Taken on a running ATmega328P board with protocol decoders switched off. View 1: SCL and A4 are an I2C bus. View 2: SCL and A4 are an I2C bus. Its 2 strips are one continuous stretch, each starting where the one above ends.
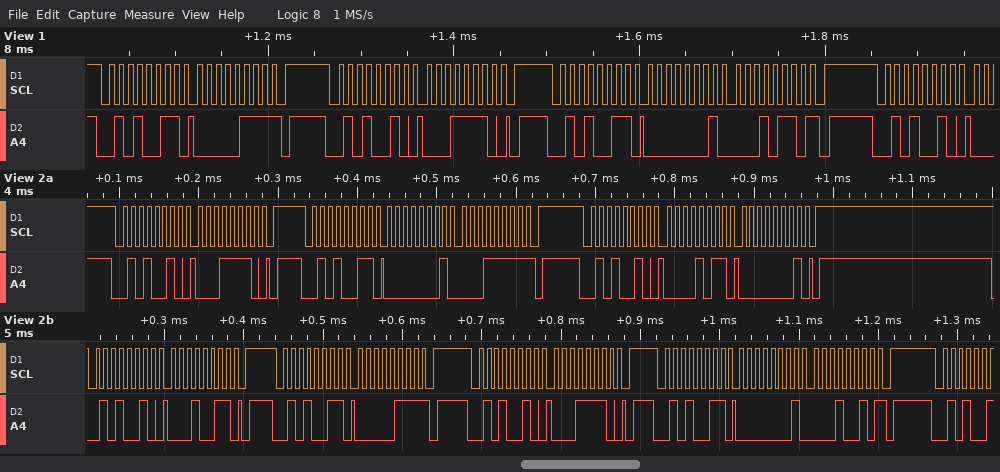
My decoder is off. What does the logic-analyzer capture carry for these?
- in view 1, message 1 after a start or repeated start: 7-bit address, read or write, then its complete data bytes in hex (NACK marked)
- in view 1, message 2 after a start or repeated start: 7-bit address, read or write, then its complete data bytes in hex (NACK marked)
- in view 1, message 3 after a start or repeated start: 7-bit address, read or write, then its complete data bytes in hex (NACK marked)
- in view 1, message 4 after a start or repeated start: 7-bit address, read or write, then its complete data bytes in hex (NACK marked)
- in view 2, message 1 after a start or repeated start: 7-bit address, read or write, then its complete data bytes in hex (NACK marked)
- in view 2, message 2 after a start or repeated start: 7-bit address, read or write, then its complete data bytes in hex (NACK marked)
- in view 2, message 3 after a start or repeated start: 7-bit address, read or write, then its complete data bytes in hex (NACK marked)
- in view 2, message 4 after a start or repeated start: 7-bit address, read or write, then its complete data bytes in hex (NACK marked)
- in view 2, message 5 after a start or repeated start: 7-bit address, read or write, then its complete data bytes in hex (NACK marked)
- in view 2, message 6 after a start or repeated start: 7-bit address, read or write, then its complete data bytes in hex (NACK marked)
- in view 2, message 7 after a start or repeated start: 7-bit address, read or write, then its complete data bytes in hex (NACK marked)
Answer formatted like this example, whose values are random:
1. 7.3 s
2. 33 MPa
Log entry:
1. 0x29 read: 07 NACK
2. 0x29 write: 1E
3. 0x29 read: 01 16 NACK
4. 0x29 write
5. 0x29 write: 1E
6. 0x29 read: 01 1F NACK
7. 0x29 write: 0B 01
8. 0x29 write: 13
9. 0x29 read: 07 NACK
10. 0x29 write: 1E
11. 0x29 read: 01 12 NACK
